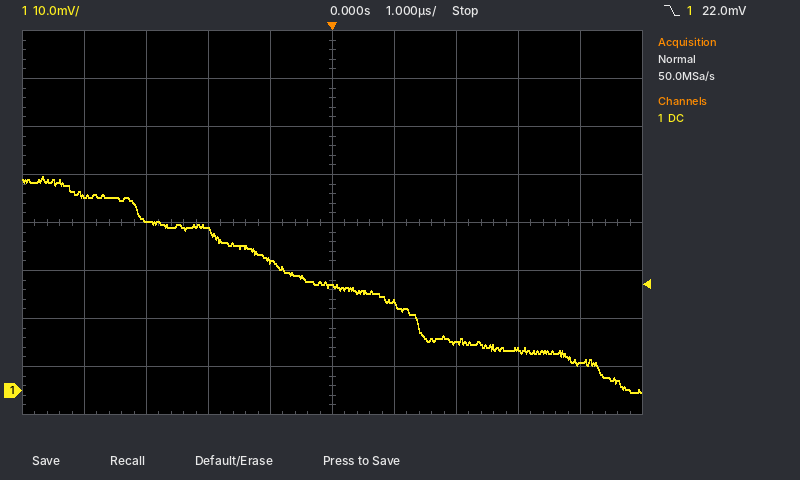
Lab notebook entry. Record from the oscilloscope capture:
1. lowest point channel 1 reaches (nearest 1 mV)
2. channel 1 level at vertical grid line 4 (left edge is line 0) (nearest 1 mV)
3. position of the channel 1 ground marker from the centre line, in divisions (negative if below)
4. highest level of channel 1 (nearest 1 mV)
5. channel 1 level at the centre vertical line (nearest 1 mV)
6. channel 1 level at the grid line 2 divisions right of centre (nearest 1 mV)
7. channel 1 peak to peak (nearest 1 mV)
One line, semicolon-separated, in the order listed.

0 mV; 27 mV; -3.5 div; 45 mV; 22 mV; 10 mV; 45 mV
